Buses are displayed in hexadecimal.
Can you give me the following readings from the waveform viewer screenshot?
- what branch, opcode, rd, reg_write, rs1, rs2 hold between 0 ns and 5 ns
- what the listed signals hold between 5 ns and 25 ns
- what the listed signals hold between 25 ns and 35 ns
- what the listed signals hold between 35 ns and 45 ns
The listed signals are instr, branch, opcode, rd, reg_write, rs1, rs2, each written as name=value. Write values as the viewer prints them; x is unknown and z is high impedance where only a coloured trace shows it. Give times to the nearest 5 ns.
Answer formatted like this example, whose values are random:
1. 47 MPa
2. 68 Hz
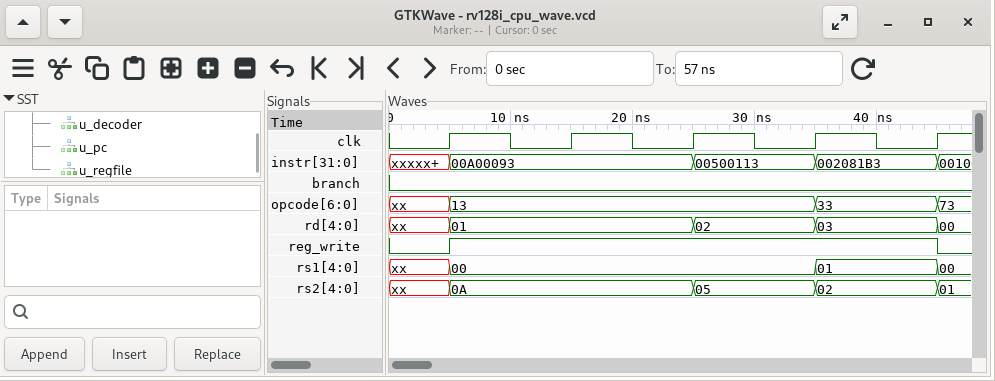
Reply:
1. branch=0, opcode=xx, rd=xx, reg_write=0, rs1=xx, rs2=xx
2. instr=00A00093, branch=0, opcode=13, rd=01, reg_write=1, rs1=00, rs2=0A
3. instr=00500113, branch=0, opcode=13, rd=02, reg_write=1, rs1=00, rs2=05
4. instr=002081B3, branch=0, opcode=33, rd=03, reg_write=1, rs1=01, rs2=02
